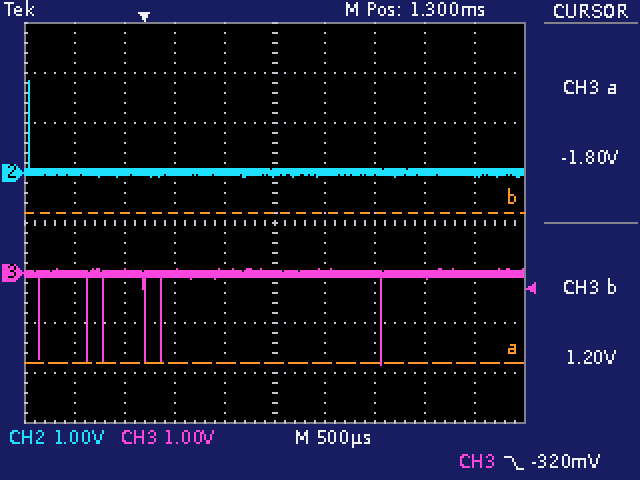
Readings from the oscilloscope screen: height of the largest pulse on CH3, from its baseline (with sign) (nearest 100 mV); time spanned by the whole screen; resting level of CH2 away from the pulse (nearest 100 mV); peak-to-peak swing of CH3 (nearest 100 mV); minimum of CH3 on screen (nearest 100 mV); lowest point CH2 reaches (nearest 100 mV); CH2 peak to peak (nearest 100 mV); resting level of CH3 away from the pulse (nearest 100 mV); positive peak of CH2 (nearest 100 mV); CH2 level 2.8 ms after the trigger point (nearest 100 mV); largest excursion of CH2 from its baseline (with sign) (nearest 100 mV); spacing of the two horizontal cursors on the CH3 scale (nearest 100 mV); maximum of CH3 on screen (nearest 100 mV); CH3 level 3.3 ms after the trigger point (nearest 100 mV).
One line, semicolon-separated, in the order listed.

-1.8 V; 5 ms; 0.0 V; 1.9 V; -1.8 V; -100 mV; 1.9 V; 0.0 V; 1.8 V; 0.0 V; +1.8 V; 3.0 V; 100 mV; 0.0 V
